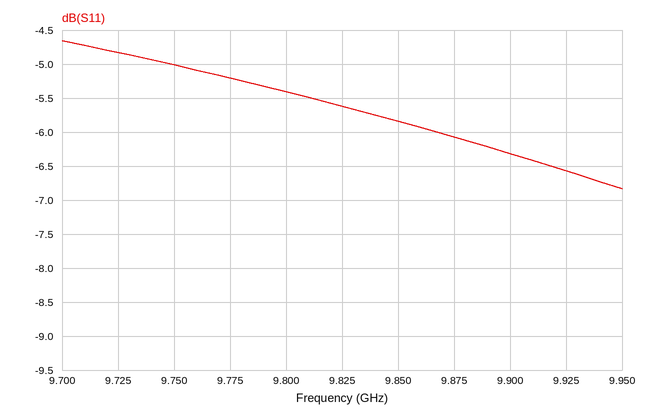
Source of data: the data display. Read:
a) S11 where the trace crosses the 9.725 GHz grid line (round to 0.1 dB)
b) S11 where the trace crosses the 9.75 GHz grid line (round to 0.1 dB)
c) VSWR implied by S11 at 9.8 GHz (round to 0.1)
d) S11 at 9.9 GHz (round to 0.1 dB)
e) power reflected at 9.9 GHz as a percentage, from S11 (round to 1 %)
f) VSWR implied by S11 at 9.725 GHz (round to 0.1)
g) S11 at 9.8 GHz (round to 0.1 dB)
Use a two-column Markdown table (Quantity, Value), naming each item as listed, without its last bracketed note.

| Quantity | Value |
|---|---|
| S11 where the trace crosses the 9.725 GHz grid line | -4.8 dB |
| S11 where the trace crosses the 9.75 GHz grid line | -5.0 dB |
| VSWR implied by S11 at 9.8 GHz | 3.3 |
| S11 at 9.9 GHz | -6.3 dB |
| power reflected at 9.9 GHz as a percentage, from S11 | 23 % |
| VSWR implied by S11 at 9.725 GHz | 3.7 |
| S11 at 9.8 GHz | -5.4 dB |
